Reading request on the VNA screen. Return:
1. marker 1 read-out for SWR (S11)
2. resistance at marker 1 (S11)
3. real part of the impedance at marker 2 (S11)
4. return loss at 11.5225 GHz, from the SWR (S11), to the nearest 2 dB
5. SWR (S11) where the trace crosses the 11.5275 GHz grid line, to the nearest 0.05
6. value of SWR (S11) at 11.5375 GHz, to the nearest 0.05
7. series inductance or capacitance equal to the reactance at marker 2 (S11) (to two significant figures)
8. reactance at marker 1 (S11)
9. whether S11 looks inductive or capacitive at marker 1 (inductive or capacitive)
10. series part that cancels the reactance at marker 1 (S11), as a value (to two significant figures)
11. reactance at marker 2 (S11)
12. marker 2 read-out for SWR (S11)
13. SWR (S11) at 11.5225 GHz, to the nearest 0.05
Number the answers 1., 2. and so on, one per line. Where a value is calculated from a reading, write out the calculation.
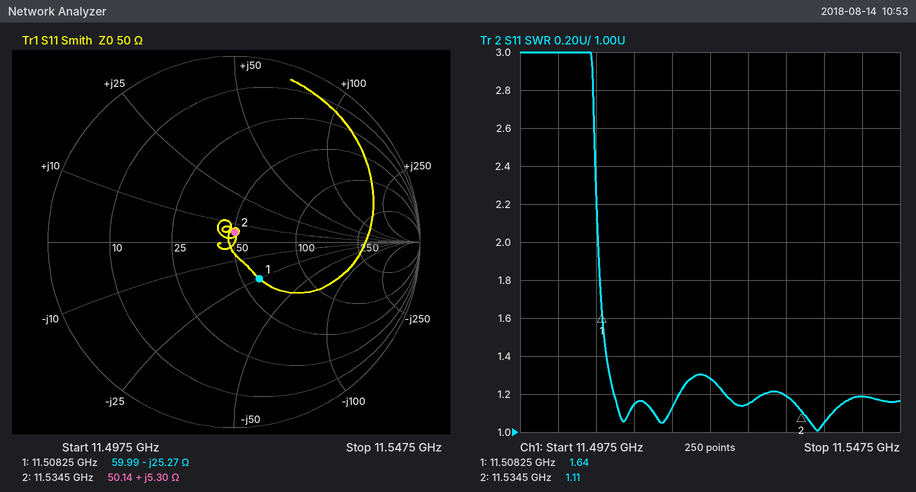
1. 1.64
2. 59.99 Ω
3. 50.14 Ω
4. −20 log10((1.3 − 1)/(1.3 + 1)) ≈ 18 dB
5. 1.15
6. 1.05
7. L = 5.3 Ω/(2π × 11.5345 GHz) ≈ 73 pH
8. -25.27 Ω
9. capacitive
10. L = 25.27 Ω/(2π × 11.50825 GHz) ≈ 349 pH, so 350 pH to two significant figures
11. +5.30 Ω
12. 1.11
13. 1.30
